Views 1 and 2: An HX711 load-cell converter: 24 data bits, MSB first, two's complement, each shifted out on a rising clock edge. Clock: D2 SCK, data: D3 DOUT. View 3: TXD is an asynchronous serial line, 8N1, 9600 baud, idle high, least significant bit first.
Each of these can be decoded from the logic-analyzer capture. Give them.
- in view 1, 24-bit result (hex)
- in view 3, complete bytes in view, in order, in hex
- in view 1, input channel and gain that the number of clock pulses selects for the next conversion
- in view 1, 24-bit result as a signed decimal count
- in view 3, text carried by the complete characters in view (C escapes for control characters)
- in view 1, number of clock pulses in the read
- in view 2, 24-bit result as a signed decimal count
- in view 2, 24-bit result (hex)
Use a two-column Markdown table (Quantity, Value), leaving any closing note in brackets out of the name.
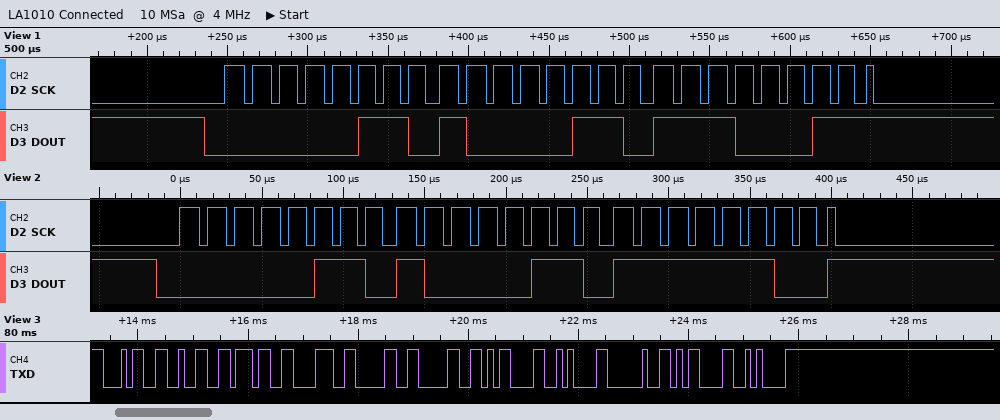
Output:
| Quantity | Value |
|---|---|
| in view 1, 24-bit result | 0x0686E3 |
| in view 3, complete bytes in view, in order, in hex | 34 32 37 38 30 30 0D 0A 20 0D 0A |
| in view 1, input channel and gain that the number of clock pulses selects for the next conversion | channel A, gain 128 |
| in view 1, 24-bit result as a signed decimal count | 427747 |
| in view 3, text carried by the complete characters in view | "427800\r\n \r\n" |
| in view 1, number of clock pulses in the read | 25 |
| in view 2, 24-bit result as a signed decimal count | 427772 |
| in view 2, 24-bit result | 0x0686FC |
